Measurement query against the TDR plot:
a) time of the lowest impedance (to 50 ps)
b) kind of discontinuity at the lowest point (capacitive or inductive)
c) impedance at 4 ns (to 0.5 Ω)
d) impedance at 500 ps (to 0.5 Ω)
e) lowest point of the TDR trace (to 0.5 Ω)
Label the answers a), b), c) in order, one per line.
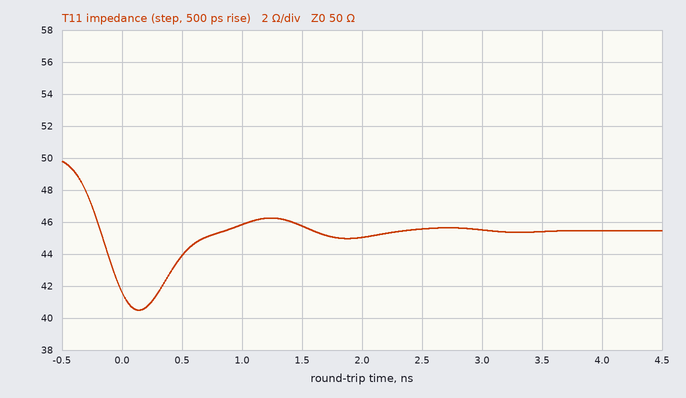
a) 150 ps
b) capacitive
c) 45.5 Ω
d) 44.0 Ω
e) 40.5 Ω
